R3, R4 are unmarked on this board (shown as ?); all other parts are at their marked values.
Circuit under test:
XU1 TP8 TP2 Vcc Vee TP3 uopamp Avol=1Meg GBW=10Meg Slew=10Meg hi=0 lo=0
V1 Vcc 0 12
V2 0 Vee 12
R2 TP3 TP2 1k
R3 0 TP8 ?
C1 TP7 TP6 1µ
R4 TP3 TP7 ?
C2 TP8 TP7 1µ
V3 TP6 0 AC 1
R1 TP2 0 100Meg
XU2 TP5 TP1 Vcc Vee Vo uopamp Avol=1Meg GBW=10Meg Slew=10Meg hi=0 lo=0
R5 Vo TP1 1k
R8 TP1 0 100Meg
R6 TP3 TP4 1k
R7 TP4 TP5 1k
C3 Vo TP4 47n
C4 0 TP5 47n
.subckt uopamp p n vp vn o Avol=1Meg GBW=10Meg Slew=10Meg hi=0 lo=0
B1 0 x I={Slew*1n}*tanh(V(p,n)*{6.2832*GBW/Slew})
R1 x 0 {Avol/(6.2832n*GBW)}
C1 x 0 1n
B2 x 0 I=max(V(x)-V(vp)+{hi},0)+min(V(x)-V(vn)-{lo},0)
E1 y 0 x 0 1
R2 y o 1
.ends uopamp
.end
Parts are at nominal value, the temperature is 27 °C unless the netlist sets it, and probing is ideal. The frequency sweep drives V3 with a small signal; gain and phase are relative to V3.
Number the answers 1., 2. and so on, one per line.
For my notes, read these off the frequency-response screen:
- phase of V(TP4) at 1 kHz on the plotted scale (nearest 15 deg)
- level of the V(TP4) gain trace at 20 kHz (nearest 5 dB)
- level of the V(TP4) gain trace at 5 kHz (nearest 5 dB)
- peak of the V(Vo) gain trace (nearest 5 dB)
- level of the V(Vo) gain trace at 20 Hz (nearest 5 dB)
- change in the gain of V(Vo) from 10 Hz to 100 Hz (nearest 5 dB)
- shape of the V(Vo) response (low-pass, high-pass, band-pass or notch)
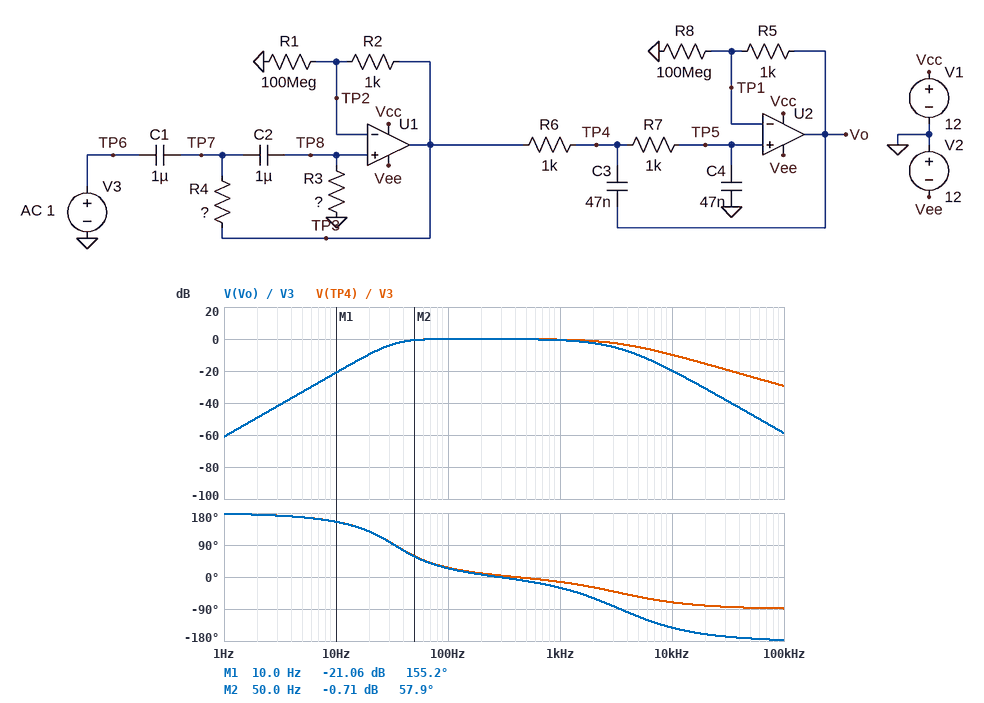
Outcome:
1. -15 deg
2. -15 dB
3. -5 dB
4. 0 dB
5. -10 dB
6. 20 dB
7. band-pass
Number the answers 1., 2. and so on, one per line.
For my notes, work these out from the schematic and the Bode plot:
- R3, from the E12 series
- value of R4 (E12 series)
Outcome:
1. 6.8 kΩ
2. 3.3 kΩ
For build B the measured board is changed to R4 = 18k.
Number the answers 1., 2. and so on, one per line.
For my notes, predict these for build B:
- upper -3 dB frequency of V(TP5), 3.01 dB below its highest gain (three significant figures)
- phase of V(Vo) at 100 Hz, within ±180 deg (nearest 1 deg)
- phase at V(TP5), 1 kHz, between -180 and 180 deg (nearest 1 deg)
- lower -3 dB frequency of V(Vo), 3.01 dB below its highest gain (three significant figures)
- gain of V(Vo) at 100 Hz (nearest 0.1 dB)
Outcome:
1. 2.24 kHz
2. 22 deg
3. -30 deg
4. 41.0 Hz
5. -0.7 dB
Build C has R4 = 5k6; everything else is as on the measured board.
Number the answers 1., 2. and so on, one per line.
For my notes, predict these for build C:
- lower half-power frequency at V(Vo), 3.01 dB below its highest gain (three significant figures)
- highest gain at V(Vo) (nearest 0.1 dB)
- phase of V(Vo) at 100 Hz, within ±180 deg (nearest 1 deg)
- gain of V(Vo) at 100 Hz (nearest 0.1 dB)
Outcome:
1. 34.3 Hz
2. -0.1 dB
3. 23 deg
4. -0.4 dB
